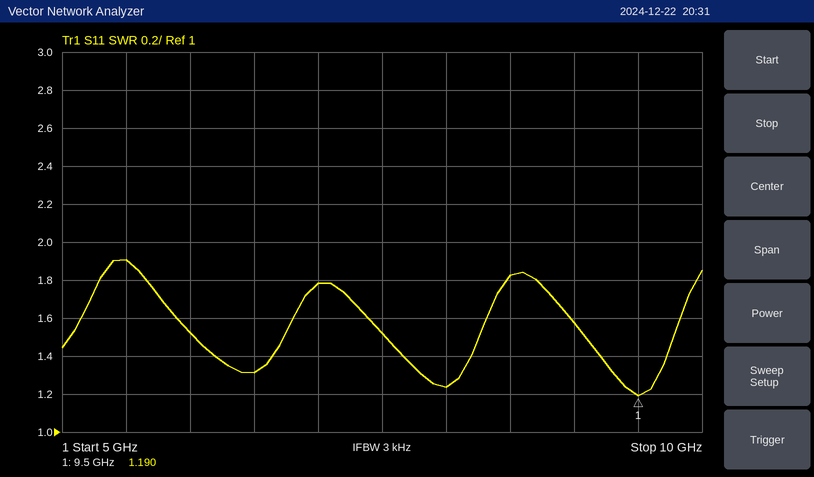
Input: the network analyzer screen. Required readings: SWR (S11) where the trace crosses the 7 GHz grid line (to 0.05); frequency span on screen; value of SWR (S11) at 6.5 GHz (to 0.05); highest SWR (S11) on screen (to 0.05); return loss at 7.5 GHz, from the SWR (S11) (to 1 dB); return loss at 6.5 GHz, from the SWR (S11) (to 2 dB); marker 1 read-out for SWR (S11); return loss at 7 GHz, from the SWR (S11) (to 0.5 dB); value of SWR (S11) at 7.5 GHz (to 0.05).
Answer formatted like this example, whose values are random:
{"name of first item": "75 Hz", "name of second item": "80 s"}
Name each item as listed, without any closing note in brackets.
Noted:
{"SWR (S11) where the trace crosses the 7 GHz grid line": "1.80", "frequency span on screen": "5 GHz", "value of SWR (S11) at 6.5 GHz": "1.30", "highest SWR (S11) on screen": "1.90", "return loss at 7.5 GHz, from the SWR (S11)": "14 dB", "return loss at 6.5 GHz, from the SWR (S11)": "18 dB", "marker 1 read-out for SWR": "1.190", "return loss at 7 GHz, from the SWR (S11)": "11.0 dB", "value of SWR (S11) at 7.5 GHz": "1.50"}
